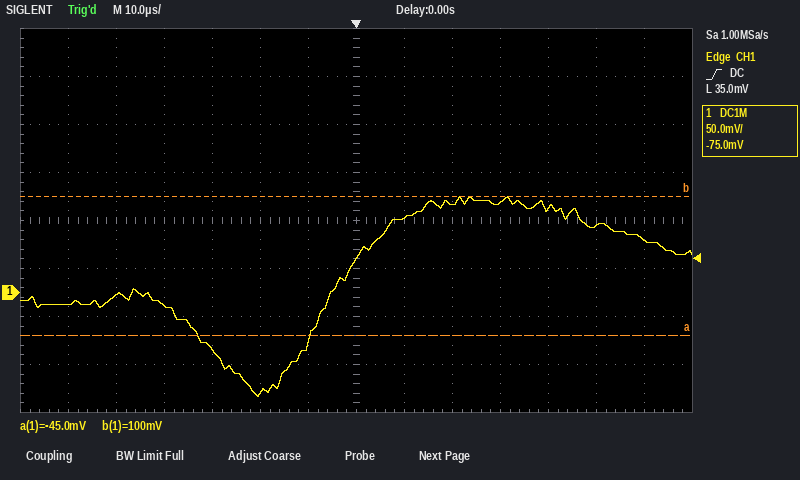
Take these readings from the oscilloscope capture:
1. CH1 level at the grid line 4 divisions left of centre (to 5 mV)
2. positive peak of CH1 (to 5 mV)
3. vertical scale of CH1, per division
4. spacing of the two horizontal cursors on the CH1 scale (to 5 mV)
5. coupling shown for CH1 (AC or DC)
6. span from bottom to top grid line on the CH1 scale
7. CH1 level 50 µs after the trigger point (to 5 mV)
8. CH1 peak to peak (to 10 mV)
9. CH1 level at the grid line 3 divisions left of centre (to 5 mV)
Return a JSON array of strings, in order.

["-15 mV", "100 mV", "50 mV", "145 mV", "DC", "400 mV", "70 mV", "210 mV", "-60 mV"]
